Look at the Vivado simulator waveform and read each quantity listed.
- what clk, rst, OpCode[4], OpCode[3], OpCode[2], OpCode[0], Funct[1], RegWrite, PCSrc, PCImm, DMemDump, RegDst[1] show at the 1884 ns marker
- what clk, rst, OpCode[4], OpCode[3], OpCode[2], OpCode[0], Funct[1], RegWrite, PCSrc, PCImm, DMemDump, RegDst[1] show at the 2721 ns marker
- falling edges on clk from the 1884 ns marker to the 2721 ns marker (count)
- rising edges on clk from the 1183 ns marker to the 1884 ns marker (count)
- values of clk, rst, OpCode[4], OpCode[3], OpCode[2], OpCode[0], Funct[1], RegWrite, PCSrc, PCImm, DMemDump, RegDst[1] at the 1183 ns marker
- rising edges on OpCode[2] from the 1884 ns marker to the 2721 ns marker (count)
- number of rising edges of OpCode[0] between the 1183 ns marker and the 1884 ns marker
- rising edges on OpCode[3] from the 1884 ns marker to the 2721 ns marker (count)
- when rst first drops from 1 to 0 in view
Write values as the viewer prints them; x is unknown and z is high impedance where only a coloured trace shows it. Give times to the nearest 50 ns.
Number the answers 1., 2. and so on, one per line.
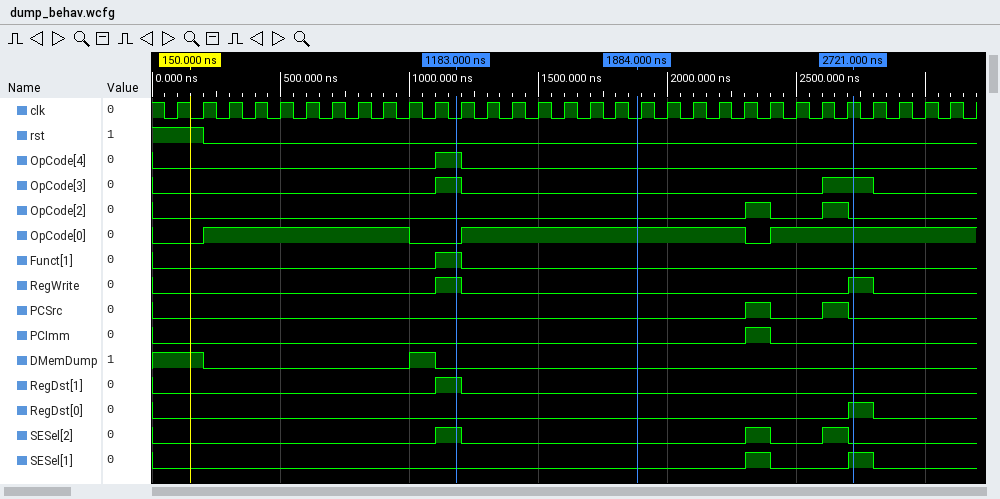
1. clk=0, rst=0, OpCode[4]=0, OpCode[3]=0, OpCode[2]=0, OpCode[0]=1, Funct[1]=0, RegWrite=0, PCSrc=0, PCImm=0, DMemDump=0, RegDst[1]=0
2. clk=1, rst=0, OpCode[4]=0, OpCode[3]=1, OpCode[2]=0, OpCode[0]=1, Funct[1]=0, RegWrite=1, PCSrc=0, PCImm=0, DMemDump=0, RegDst[1]=0
3. 8
4. 7
5. clk=0, rst=0, OpCode[4]=1, OpCode[3]=1, OpCode[2]=0, OpCode[0]=0, Funct[1]=1, RegWrite=1, PCSrc=0, PCImm=0, DMemDump=0, RegDst[1]=1
6. 2
7. 1
8. 1
9. 200 ns
